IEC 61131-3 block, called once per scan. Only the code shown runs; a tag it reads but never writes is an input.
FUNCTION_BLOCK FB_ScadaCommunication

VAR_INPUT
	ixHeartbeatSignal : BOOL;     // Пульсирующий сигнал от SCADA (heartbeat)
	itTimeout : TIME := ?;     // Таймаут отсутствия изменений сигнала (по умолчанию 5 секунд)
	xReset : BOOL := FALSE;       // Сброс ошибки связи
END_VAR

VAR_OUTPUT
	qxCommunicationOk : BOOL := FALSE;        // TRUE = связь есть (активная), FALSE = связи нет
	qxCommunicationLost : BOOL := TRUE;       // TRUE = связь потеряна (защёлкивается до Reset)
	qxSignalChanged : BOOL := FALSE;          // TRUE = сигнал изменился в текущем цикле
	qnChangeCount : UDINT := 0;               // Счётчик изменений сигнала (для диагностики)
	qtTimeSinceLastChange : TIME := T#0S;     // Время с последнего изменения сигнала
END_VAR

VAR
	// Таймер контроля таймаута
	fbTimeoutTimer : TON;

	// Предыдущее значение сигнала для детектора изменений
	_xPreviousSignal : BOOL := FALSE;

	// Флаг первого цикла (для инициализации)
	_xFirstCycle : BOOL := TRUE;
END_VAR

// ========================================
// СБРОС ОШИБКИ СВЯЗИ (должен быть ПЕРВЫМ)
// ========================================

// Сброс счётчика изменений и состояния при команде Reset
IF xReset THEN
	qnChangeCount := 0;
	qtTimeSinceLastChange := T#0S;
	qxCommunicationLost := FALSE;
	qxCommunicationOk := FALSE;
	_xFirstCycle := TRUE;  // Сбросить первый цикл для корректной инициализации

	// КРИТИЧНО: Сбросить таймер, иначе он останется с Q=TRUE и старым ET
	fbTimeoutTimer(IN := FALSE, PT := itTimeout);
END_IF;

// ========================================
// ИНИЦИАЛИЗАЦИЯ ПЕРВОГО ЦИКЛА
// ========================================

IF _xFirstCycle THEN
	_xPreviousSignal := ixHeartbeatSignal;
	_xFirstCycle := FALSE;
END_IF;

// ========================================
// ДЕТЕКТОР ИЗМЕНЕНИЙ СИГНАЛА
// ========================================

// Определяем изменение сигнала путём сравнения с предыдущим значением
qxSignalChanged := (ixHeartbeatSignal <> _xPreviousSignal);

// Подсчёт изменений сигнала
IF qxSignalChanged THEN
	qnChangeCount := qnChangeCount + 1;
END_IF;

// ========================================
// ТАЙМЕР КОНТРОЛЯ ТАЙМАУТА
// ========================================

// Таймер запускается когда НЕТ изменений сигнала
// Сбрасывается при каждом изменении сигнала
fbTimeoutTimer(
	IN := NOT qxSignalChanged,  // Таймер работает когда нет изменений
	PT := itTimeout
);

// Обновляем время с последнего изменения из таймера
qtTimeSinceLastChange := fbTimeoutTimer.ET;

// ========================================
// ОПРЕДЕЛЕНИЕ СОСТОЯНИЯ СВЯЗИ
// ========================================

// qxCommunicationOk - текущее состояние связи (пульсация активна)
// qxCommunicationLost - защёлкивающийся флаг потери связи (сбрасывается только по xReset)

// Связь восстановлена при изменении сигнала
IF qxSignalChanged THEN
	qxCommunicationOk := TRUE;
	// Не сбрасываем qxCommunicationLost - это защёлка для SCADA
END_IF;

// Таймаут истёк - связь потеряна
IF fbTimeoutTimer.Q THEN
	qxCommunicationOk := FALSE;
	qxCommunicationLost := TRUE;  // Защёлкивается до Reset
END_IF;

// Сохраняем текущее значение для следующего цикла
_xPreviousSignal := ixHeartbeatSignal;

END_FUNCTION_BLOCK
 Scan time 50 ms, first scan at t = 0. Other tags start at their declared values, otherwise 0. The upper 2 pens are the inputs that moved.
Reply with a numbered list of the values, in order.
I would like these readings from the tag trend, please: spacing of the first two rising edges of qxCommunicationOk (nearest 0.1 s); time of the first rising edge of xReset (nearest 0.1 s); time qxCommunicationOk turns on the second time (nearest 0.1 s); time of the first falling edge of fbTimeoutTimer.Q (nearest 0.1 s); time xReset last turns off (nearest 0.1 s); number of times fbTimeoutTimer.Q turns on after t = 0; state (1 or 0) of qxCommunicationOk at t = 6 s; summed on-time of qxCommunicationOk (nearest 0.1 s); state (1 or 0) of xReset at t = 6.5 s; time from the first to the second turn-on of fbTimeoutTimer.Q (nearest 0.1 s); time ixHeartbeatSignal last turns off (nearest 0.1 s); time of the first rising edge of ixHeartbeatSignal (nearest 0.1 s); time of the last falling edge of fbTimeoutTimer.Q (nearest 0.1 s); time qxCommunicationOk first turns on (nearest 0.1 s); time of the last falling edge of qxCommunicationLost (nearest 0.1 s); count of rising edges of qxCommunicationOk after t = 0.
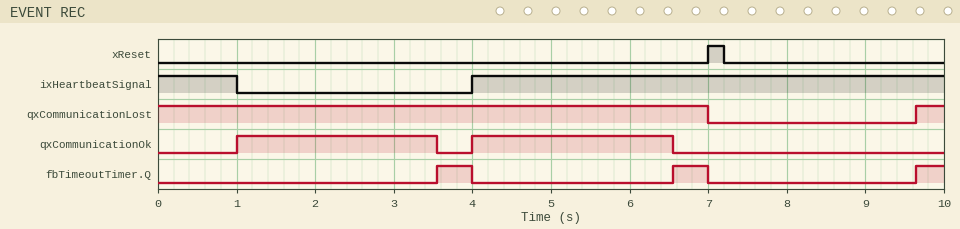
1. 3.0 s
2. 7.0 s
3. 4.0 s
4. 4.0 s
5. 7.2 s
6. 3
7. 1
8. 5.1 s
9. 0
10. 3.0 s
11. 1.0 s
12. 4.0 s
13. 7.0 s
14. 1.0 s
15. 7.0 s
16. 2
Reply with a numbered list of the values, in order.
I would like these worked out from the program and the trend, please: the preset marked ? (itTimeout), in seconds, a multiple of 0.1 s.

1. 2.5 s
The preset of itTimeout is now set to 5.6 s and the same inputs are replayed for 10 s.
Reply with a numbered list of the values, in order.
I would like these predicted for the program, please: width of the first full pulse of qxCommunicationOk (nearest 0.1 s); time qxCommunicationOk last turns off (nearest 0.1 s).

1. 6.0 s
2. 7.0 s
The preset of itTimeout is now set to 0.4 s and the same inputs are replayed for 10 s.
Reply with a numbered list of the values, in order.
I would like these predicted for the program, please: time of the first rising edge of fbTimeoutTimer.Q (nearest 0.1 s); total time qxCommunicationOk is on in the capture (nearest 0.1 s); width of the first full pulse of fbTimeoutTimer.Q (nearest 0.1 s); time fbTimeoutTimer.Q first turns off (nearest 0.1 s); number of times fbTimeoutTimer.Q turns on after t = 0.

1. 0.4 s
2. 0.9 s
3. 0.6 s
4. 1.0 s
5. 4
